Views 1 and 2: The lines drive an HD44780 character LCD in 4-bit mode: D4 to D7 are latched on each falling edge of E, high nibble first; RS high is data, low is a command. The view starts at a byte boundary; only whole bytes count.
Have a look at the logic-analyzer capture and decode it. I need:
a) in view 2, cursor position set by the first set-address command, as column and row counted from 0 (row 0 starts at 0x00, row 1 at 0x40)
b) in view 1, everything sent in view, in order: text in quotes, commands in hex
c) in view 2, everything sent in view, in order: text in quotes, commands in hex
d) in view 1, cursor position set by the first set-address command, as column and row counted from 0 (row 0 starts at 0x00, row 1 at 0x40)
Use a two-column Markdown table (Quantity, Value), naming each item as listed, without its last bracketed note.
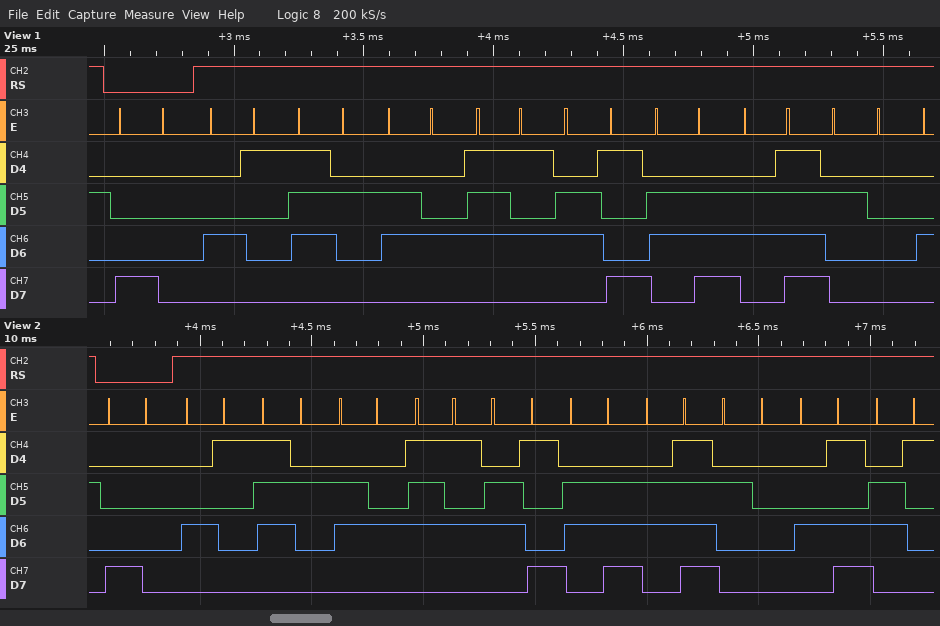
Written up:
| Quantity | Value |
|---|---|
| in view 2, cursor position set by the first set-address command, as column and row counted from 0 | column 0, row 0 |
| in view 1, everything sent in view, in order: text in quotes, commands in hex | 0x80 "Arduino " |
| in view 2, everything sent in view, in order: text in quotes, commands in hex | 0x80 "Arduino Ma" |
| in view 1, cursor position set by the first set-address command, as column and row counted from 0 | column 0, row 0 |
